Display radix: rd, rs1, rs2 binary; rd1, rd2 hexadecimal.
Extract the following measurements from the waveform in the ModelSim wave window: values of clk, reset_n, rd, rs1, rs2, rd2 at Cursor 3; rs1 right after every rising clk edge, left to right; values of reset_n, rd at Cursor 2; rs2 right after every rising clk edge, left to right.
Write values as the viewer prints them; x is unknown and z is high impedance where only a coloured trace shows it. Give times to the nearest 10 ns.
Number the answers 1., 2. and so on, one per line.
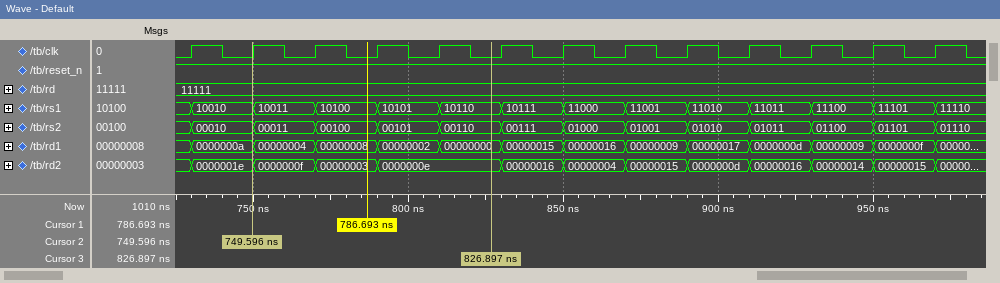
1. clk=0, reset_n=1, rd=11111, rs1=10110, rs2=00110, rd2=0000000e
2. 10010, 10011, 10100, 10101, 10110, 10111, 11000, 11001, 11010, 11011, 11100, 11101, 11110
3. reset_n=1, rd=11111
4. 00010, 00011, 00100, 00101, 00110, 00111, 01000, 01001, 01010, 01011, 01100, 01101, 01110
